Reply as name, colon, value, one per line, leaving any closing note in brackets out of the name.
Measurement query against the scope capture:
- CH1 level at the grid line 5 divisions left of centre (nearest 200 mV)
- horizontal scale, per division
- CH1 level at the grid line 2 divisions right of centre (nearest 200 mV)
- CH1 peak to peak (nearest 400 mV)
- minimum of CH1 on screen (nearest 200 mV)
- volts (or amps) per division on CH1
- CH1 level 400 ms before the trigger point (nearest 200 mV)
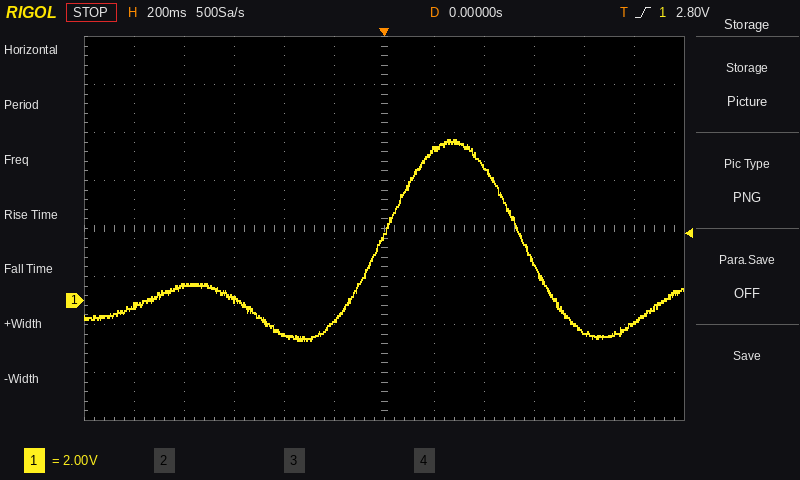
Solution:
CH1 level at the grid line 5 divisions left of centre: -200 mV
horizontal scale, per division: 200 ms
CH1 level at the grid line 2 divisions right of centre: 5.6 V
CH1 peak to peak: 8.4 V
minimum of CH1 on screen: -1.6 V
volts (or amps) per division on CH1: 2 V
CH1 level 400 ms before the trigger point: -1.4 V
